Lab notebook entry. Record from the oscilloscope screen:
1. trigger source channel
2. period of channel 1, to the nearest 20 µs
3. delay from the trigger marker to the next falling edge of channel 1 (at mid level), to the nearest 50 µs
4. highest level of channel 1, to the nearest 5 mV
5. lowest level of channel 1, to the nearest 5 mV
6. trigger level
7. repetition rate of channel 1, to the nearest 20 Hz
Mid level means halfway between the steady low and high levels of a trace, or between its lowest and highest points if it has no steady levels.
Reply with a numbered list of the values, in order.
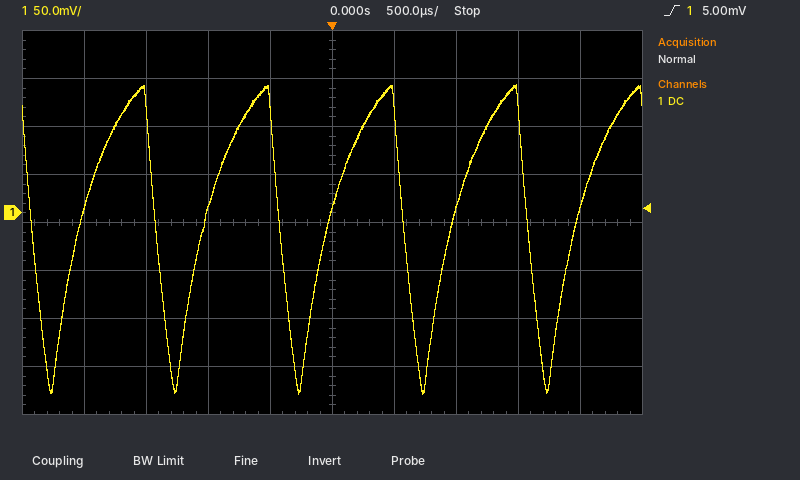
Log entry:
1. channel 1
2. 1.00 ms
3. 600 µs
4. 135 mV
5. -190 mV
6. 5.00 mV
7. 1.00 kHz
